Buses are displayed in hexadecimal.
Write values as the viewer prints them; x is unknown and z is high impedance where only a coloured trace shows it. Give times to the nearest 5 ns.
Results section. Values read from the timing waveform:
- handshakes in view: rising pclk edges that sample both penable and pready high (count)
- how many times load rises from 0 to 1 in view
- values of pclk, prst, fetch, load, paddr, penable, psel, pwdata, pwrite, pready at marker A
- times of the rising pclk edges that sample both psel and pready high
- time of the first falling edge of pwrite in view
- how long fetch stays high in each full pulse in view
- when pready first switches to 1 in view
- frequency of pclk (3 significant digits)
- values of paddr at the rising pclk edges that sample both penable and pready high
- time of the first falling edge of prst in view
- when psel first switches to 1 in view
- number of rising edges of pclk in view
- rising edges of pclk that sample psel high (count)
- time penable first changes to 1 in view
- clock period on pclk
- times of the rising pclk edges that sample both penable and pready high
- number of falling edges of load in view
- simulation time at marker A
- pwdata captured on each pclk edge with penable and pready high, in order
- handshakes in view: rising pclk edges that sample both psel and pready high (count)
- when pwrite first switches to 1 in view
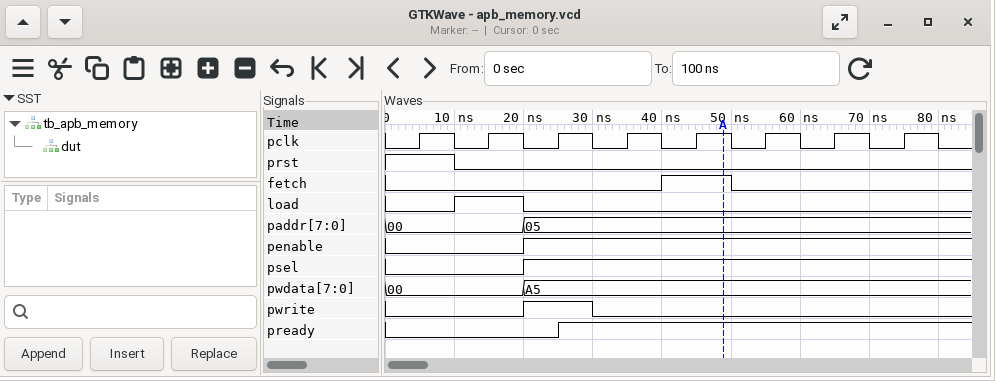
5
1
pclk=1, prst=0, fetch=1, load=0, paddr=05, penable=1, psel=1, pwdata=A5, pwrite=0, pready=1
35 ns, 45 ns, 55 ns, 65 ns, 75 ns
30 ns
10 ns
25 ns
100 MHz
05, 05, 05, 05, 05
10 ns
20 ns
8
6
20 ns
10 ns
35 ns, 45 ns, 55 ns, 65 ns, 75 ns
1
50 ns
A5, A5, A5, A5, A5
5
20 ns
